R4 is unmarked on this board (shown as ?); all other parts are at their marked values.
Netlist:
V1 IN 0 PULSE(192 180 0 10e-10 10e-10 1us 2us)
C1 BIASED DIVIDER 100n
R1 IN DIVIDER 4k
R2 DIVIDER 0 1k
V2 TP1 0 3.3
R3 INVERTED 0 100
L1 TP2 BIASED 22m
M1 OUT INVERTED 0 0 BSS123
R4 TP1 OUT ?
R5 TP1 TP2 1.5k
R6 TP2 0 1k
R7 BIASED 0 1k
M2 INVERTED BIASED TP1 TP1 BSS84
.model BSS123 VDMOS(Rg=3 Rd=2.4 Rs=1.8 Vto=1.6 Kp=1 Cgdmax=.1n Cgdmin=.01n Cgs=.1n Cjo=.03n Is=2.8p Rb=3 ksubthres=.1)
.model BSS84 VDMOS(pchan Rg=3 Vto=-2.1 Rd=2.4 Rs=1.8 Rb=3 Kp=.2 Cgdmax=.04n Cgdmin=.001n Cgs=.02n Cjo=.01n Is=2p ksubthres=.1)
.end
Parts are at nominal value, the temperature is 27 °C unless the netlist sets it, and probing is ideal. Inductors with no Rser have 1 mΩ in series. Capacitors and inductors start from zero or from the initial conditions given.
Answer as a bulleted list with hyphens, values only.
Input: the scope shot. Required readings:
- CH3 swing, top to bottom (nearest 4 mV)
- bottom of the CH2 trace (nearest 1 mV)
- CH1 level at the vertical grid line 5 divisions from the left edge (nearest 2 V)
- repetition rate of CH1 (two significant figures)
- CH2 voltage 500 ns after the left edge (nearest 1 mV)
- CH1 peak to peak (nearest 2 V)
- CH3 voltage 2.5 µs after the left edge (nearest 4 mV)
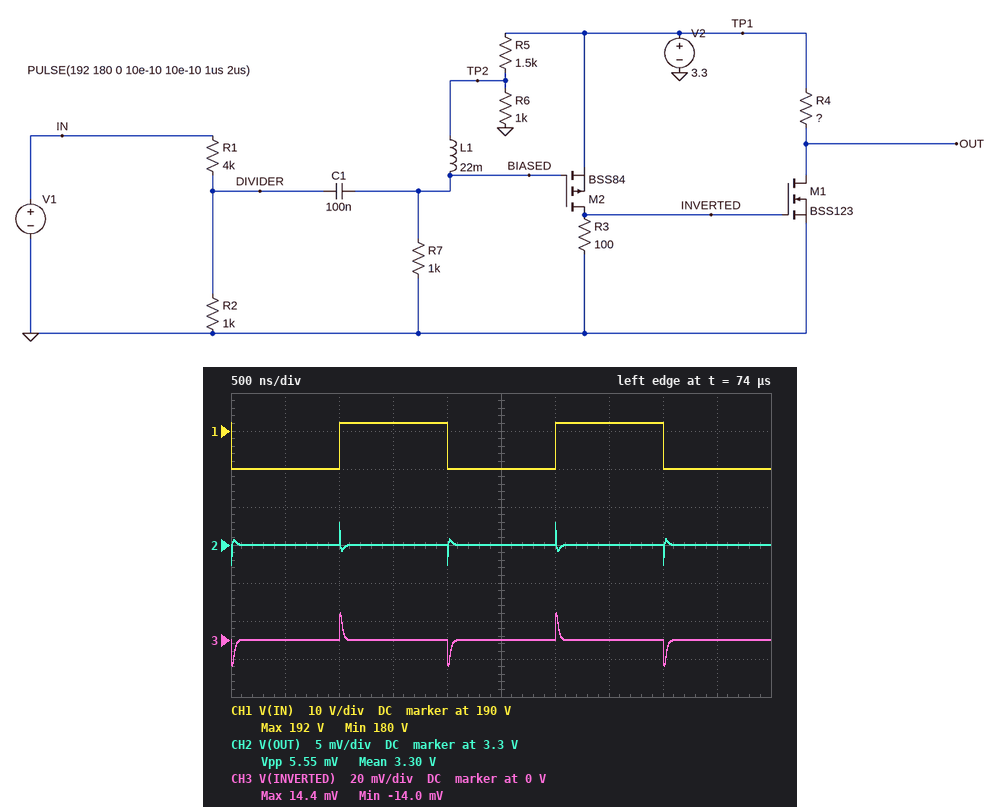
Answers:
- 28 mV
- 3.297 V
- 180 V
- 500 kHz
- 3.300 V
- 12 V
- 0 V
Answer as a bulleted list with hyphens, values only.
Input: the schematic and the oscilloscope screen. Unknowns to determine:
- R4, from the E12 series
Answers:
- 82 Ω
